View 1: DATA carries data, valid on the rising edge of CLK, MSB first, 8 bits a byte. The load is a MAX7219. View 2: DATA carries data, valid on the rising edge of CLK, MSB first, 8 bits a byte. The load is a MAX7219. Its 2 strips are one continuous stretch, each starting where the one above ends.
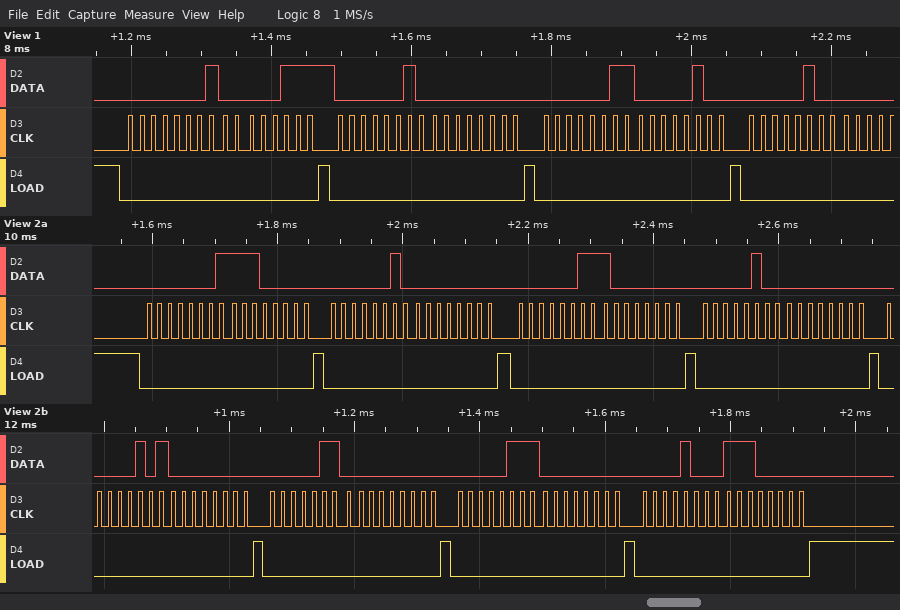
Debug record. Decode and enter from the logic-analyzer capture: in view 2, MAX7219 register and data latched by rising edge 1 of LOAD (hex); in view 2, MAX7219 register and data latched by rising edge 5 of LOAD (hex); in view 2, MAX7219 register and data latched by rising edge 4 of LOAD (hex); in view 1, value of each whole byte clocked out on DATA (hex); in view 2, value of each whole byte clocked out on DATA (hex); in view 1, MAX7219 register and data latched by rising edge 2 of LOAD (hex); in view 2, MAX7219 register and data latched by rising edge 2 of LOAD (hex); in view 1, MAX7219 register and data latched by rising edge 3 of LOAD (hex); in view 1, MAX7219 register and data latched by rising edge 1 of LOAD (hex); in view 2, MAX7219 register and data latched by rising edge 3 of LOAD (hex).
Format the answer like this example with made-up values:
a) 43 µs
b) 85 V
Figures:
a) register 0x1, data 0xE0
b) register 0x5, data 0x00
c) register 0x4, data 0x00
d) 0x01 0x07 0x02 0x00 0x03 0x04 0x04
e) 0x01 0xE0 0x02 0x00 0x03 0x80 0x04 0x00 0x05 0x00 0x06 0x00 0x07 0x00 0x08 0xE0
f) register 0x2, data 0x00
g) register 0x2, data 0x00
h) register 0x3, data 0x04
i) register 0x1, data 0x07
j) register 0x3, data 0x80
